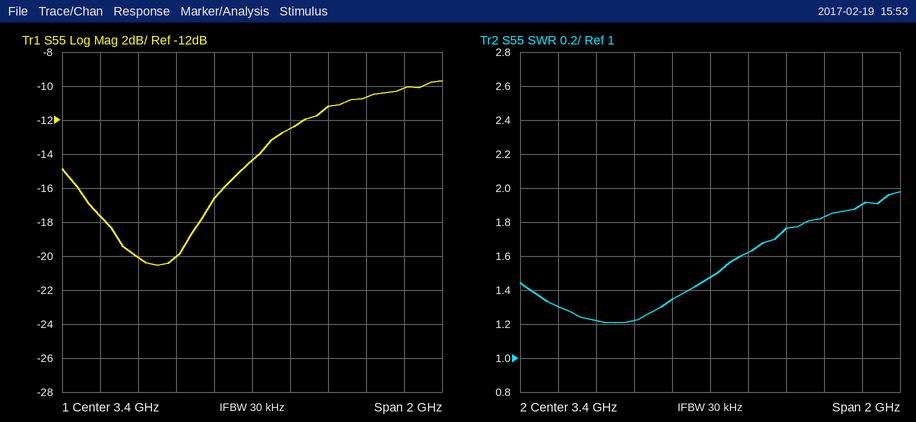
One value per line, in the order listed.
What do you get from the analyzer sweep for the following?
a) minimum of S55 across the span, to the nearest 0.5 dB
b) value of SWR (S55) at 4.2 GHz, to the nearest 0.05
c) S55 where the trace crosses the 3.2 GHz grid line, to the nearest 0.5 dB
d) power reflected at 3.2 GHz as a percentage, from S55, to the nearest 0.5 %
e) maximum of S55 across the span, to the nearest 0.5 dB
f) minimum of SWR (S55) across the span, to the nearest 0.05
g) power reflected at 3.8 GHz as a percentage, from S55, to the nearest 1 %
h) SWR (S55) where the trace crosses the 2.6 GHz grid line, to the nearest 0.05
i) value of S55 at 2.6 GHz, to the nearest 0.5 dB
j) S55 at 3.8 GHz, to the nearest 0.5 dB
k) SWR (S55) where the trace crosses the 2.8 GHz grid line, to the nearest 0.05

-20.5 dB
1.90
-16.5 dB
2.0 %
-9.5 dB
1.20
8 %
1.30
-17.5 dB
-11.0 dB
1.20
